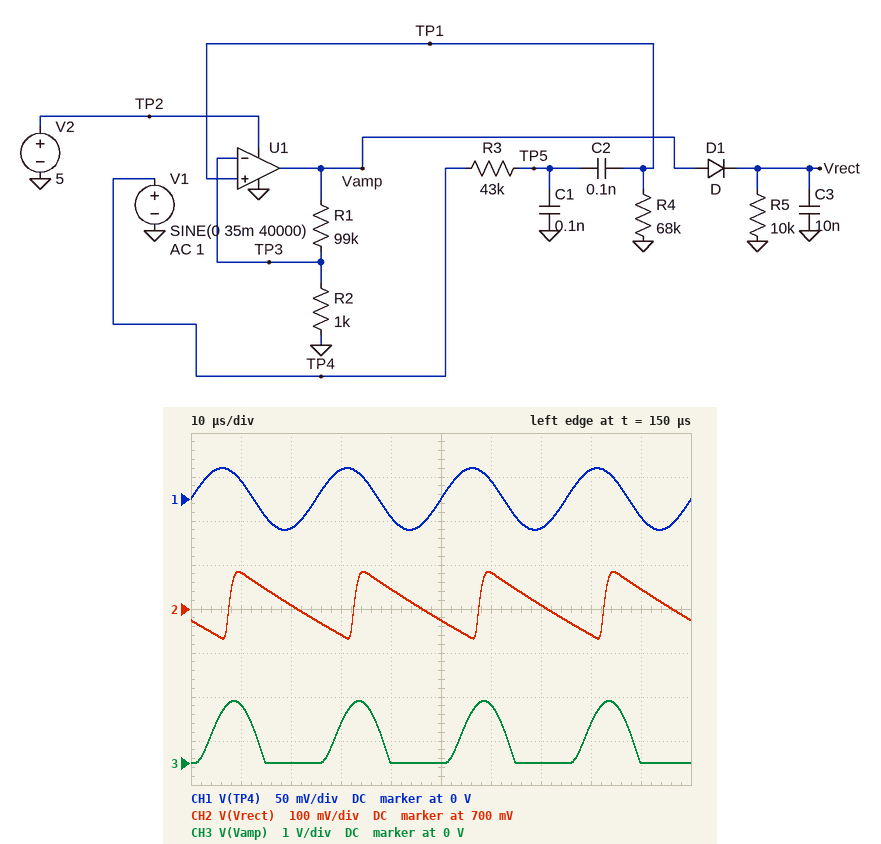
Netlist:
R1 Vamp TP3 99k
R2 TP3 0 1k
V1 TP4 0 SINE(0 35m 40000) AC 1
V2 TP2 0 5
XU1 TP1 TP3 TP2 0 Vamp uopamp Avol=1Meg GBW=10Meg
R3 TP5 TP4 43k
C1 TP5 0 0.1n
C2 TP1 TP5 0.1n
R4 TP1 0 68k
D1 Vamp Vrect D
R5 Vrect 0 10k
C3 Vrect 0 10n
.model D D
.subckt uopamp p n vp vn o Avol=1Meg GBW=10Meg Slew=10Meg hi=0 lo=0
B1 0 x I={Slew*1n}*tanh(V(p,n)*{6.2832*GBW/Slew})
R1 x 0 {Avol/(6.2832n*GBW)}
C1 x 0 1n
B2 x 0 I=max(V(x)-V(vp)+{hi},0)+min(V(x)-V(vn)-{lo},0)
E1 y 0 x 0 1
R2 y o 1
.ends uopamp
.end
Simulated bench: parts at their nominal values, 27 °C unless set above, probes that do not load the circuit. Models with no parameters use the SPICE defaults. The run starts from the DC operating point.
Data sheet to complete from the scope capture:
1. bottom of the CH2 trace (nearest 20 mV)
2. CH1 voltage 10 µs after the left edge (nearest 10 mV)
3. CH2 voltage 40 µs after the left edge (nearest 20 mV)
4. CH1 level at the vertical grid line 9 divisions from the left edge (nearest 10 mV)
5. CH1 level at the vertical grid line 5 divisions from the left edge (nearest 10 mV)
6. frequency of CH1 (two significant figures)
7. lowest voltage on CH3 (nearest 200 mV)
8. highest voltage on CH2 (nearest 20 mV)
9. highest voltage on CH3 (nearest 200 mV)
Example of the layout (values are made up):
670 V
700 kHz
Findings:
640 mV
20 mV
740 mV
-20 mV
0 V
40 kHz
0 V
780 mV
1.4 V
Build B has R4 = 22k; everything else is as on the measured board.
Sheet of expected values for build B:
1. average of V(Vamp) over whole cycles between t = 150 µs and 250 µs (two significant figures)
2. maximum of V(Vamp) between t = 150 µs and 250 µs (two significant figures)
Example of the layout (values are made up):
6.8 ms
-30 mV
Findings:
220 mV
660 mV
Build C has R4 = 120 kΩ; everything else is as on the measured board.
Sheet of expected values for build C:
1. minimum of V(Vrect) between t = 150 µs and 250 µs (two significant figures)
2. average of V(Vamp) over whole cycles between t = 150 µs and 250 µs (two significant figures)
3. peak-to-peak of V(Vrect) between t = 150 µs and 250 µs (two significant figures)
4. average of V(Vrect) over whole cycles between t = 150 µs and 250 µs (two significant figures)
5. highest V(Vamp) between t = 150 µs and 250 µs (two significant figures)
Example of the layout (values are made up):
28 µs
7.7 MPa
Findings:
900 mV
570 mV
220 mV
1.0 V
1.7 V
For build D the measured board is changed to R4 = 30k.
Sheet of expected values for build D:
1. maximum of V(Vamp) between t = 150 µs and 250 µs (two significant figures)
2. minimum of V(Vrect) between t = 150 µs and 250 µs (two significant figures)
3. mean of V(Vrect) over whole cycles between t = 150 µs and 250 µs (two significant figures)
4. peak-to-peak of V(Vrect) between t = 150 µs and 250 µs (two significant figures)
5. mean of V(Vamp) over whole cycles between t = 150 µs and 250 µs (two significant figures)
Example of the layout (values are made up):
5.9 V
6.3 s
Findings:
840 mV
190 mV
210 mV
45 mV
280 mV
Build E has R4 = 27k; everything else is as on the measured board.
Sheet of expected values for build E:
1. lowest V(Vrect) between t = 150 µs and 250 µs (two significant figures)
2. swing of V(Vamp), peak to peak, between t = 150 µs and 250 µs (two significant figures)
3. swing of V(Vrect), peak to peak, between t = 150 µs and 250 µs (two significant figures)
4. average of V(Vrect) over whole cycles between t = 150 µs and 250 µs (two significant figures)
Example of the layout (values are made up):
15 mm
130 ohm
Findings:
140 mV
780 mV
33 mV
160 mV
